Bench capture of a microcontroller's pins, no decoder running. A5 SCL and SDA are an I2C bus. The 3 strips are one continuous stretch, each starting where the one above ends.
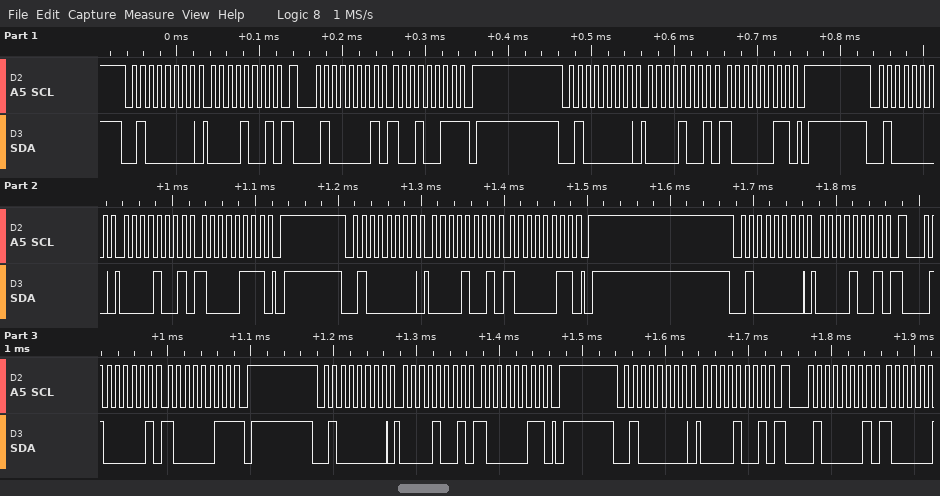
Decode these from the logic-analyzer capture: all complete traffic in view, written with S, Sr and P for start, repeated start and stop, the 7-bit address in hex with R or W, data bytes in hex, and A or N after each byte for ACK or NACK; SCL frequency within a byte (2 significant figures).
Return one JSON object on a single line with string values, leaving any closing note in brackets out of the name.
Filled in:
{"all complete traffic in view, written with S, Sr and P for start, repeated start and stop, the 7-bit address in hex with R or W, data bytes in hex, and A or N after each byte for ACK or NACK": "S 20W A 09 A Sr 20R A 93 N P S 20W A 09 A 83 A P S 20W A 09 A 87 A P S 20W A 09 A 83 A P S 20W A 09 A Sr 20R A 83 N P S 20W A 09 A 83 A P S 20W A 09 A Sr 20R A", "SCL frequency within a byte": "100 kHz"}
